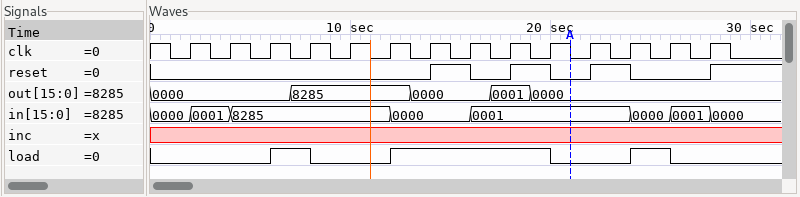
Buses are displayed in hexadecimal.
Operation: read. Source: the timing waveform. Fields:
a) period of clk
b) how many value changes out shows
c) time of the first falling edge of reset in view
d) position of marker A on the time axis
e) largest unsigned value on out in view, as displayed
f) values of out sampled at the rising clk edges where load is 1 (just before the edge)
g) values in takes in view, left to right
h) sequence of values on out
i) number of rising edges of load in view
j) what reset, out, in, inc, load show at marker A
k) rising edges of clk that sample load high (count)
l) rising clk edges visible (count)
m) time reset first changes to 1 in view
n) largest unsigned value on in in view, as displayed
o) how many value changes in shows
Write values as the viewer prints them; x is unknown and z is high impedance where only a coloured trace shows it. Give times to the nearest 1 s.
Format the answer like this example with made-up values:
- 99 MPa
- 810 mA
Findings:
- 2 s
- 4
- 16 s
- 21 s
- 8285
- 8285, 0000, 0000, 0001, 0000, 0000
- 0000, 0001, 8285, 0000, 0001, 0000, 0001, 0000
- 0000, 8285, 0000, 0001, 0000
- 3
- reset=0, out=0000, in=0001, inc=x, load=0
- 6
- 14
- 14 s
- 8285
- 7
